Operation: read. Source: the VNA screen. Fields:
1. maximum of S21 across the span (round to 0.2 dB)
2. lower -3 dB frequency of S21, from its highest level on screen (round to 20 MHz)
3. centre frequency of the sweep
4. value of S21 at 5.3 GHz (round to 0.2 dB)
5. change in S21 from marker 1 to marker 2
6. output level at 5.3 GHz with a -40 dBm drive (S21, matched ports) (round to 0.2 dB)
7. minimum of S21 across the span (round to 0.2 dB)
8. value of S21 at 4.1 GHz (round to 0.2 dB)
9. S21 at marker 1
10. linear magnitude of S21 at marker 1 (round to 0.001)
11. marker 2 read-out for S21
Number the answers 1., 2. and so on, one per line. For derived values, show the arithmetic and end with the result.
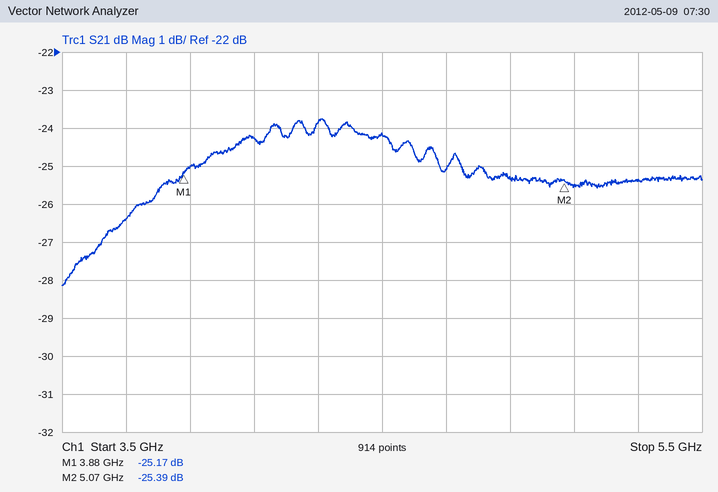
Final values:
1. -23.8 dB
2. 3.64 GHz
3. 4.5 GHz
4. -25.4 dB
5. -25.39 − (-25.17) = -0.22 dB
6. -40 dBm + (-25.4 dB) = -65.4 dBm
7. -28.2 dB
8. -24.2 dB
9. -25.17 dB
10. 10^(-25.17/20) ≈ 0.055
11. -25.39 dB
